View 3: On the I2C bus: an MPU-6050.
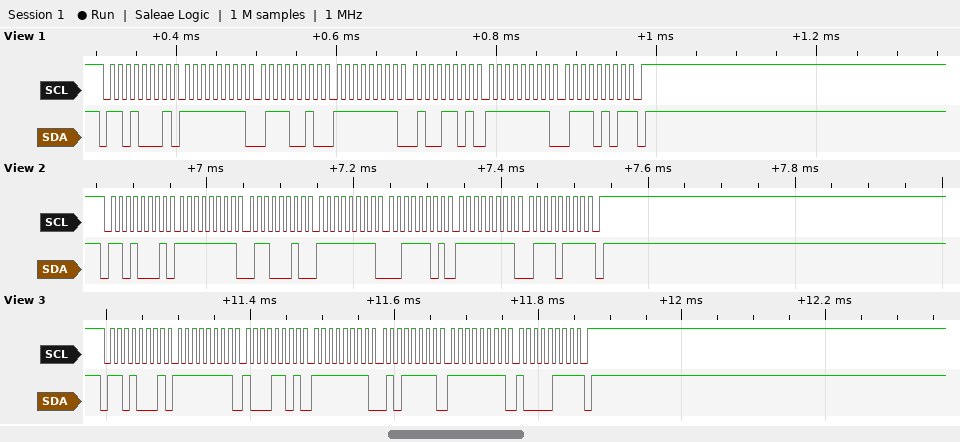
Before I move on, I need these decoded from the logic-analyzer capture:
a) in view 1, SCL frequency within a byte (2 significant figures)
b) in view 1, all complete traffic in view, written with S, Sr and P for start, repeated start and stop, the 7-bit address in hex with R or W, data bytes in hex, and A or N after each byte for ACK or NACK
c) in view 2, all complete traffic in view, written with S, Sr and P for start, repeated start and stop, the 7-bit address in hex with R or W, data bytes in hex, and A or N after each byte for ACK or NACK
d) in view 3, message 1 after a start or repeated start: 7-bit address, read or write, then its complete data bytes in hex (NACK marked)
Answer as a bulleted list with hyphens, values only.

- 100 kHz
- S 68R A FF A 72 A FF A 4D A FF A 75 N P
- S 68R A FF A 62 A FF A 3D A FF A 77 N P
- 0x68 read: FF 8D FF 5F FF 87 NACK
